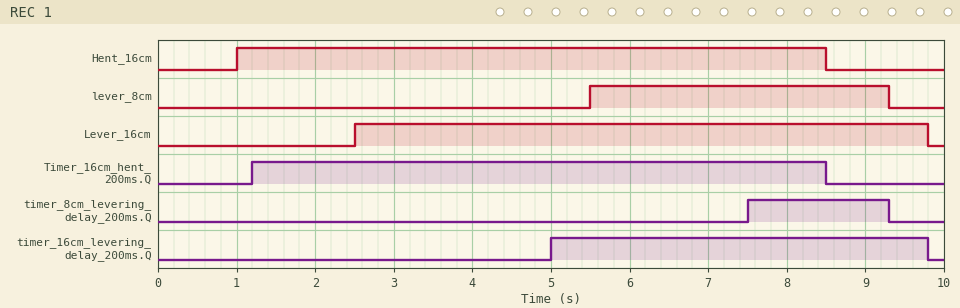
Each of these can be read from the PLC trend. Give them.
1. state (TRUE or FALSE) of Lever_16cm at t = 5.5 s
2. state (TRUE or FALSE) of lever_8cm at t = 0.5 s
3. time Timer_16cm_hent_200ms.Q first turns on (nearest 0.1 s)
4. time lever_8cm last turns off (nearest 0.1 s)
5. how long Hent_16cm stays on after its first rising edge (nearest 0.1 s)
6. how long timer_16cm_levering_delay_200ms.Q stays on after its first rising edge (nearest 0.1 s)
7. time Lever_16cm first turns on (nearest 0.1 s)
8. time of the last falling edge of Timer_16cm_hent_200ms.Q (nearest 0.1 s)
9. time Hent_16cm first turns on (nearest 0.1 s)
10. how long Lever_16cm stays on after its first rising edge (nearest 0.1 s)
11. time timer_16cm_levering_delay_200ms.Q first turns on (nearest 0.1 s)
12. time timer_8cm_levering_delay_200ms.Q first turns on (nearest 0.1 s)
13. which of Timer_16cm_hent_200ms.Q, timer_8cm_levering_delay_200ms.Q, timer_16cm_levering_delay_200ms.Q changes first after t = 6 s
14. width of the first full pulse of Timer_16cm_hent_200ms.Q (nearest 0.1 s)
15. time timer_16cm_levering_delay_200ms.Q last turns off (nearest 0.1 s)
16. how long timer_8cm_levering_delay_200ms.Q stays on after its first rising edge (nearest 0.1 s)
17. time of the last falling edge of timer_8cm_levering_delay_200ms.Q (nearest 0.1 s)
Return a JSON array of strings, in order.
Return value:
["TRUE", "FALSE", "1.2 s", "9.3 s", "7.5 s", "4.8 s", "2.5 s", "8.5 s", "1.0 s", "7.3 s", "5.0 s", "7.5 s", "timer_8cm_levering_delay_200ms.Q", "7.3 s", "9.8 s", "1.8 s", "9.3 s"]
